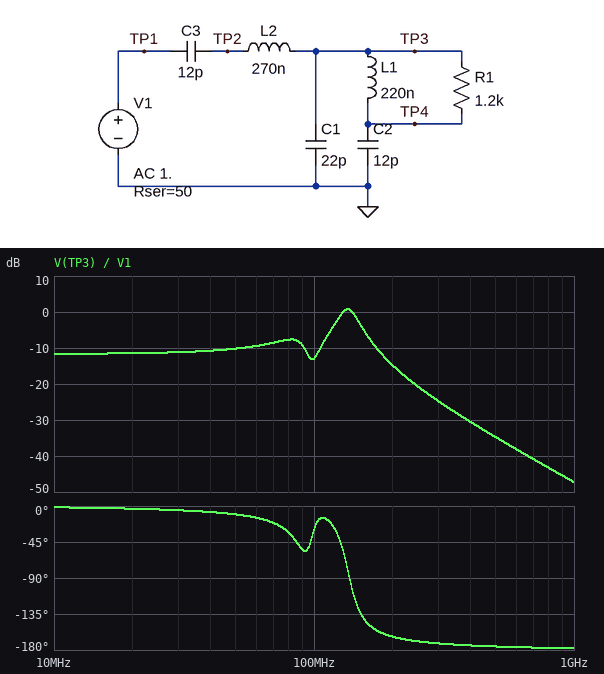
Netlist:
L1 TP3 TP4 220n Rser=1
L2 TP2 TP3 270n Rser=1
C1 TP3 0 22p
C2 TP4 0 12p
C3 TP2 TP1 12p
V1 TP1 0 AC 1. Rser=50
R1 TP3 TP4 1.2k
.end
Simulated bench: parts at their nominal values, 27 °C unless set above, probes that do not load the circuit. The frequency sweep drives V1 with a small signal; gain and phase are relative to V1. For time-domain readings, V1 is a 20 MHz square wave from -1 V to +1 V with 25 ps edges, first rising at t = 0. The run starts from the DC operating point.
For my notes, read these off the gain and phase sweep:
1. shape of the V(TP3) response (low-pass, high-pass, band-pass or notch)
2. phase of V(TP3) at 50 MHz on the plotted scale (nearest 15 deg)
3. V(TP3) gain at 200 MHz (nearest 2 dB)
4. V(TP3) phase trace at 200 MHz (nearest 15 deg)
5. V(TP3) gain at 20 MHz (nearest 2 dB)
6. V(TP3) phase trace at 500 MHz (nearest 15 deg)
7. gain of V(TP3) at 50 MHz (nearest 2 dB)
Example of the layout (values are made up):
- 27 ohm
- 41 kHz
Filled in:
- low-pass
- -15 deg
- -14 dB
- -165 deg
- -12 dB
- -180 deg
- -10 dB
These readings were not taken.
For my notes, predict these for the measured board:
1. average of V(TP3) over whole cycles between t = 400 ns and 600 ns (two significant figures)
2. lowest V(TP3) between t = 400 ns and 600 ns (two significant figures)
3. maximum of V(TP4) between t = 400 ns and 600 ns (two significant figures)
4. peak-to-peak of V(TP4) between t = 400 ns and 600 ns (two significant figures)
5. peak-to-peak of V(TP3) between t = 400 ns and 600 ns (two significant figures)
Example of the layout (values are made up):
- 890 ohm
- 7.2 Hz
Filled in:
- 260 mV
- -290 mV
- 1.3 V
- 2.1 V
- 1.1 V
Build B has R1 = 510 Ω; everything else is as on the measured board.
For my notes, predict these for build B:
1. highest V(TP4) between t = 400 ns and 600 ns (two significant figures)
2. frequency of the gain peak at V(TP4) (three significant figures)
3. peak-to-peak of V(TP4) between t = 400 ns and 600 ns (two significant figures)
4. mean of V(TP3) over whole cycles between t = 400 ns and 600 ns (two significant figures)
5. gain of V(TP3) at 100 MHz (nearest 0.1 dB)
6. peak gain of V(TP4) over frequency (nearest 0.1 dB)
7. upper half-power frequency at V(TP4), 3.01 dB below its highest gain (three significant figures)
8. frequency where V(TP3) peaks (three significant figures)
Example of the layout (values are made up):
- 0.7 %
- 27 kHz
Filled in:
- 1.2 V
- 93.2 MHz
- 1.8 V
- 260 mV
- -8.3 dB
- 3.8 dB
- 113 MHz
- 134 MHz
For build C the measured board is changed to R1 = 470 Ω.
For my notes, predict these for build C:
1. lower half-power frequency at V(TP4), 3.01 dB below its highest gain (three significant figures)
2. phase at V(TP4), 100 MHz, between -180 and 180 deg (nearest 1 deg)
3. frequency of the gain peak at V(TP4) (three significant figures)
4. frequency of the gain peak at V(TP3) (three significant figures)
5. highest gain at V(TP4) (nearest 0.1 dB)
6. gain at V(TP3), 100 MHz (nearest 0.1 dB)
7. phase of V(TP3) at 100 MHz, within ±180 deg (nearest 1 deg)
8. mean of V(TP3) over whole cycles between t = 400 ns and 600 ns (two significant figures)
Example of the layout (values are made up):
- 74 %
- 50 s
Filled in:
- 79.7 MHz
- -130 deg
- 93.2 MHz
- 133 MHz
- 3.5 dB
- -7.9 dB
- -48 deg
- 260 mV
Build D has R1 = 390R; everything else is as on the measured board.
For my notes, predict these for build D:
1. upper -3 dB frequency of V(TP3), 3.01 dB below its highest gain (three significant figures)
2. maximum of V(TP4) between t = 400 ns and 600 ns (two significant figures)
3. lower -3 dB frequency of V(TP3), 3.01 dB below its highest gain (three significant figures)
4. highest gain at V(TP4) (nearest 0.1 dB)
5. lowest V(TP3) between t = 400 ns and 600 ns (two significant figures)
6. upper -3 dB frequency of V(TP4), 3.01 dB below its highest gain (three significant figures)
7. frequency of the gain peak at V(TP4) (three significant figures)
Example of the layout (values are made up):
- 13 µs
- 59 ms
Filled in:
- 156 MHz
- 1.1 V
- 72.7 MHz
- 2.9 dB
- -260 mV
- 113 MHz
- 93.3 MHz
